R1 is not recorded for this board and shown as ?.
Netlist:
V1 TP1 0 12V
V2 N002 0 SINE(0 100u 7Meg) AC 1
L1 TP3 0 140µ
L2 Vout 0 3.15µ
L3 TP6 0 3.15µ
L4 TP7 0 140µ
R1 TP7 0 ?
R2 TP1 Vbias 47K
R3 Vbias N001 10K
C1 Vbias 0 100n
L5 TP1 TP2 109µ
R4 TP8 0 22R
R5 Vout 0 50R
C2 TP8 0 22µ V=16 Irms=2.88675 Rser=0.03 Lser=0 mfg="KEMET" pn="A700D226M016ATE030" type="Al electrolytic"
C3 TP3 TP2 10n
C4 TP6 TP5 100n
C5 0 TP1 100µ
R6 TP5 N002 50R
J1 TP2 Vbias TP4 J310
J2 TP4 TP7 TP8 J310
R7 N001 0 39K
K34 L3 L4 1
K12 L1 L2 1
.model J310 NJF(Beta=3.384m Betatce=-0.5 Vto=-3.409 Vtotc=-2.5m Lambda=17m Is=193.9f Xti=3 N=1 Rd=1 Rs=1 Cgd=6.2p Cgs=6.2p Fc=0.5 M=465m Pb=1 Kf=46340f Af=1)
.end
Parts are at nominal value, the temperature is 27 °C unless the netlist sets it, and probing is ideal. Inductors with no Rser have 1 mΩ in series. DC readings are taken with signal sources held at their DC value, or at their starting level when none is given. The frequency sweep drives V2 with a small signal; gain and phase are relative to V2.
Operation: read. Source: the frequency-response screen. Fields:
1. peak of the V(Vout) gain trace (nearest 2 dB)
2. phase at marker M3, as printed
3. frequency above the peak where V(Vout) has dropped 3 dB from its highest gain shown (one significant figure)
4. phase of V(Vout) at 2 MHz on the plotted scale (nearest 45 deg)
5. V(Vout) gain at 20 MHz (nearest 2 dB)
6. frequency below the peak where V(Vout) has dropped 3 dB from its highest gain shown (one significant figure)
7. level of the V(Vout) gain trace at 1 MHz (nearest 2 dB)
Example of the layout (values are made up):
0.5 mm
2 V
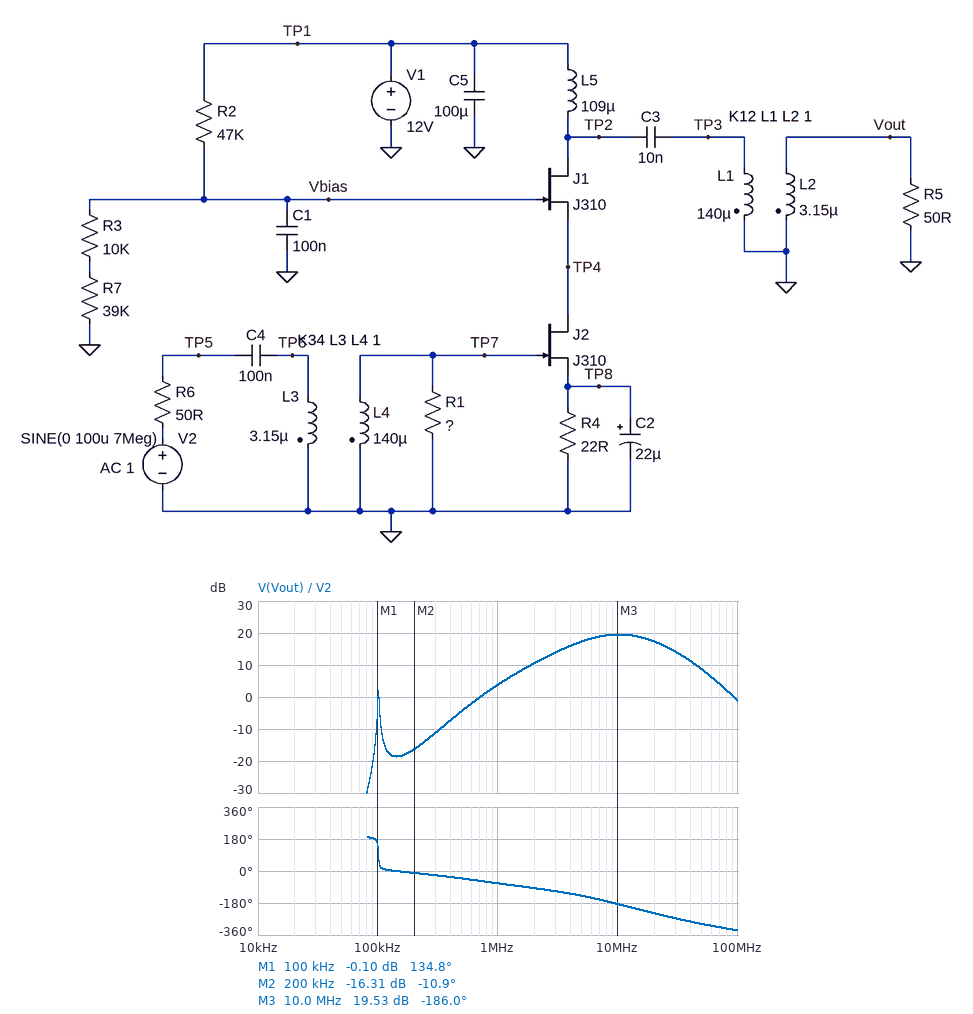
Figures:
20 dB
-186.0 deg
20 MHz
-90 deg
18 dB
4 MHz
4 dB
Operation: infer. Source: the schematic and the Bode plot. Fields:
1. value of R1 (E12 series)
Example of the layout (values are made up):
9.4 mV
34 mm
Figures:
680 Ω
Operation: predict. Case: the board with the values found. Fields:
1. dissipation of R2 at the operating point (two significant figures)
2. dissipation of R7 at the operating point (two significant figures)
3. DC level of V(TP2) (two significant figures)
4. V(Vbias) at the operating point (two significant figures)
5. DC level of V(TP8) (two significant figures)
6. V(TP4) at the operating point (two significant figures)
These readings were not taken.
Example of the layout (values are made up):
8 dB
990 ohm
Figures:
730 µW
610 µW
12 V
6.1 V
620 mV
6.7 V
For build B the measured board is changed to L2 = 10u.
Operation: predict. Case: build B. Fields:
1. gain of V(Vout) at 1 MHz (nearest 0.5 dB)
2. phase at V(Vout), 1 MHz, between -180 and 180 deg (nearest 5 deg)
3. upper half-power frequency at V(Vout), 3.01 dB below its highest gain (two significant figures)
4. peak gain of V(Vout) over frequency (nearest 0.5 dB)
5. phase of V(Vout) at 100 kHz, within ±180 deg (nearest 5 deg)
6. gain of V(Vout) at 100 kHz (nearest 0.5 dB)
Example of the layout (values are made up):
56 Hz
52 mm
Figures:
8.0 dB
-90 deg
30 MHz
15.0 dB
110 deg
-3.5 dB
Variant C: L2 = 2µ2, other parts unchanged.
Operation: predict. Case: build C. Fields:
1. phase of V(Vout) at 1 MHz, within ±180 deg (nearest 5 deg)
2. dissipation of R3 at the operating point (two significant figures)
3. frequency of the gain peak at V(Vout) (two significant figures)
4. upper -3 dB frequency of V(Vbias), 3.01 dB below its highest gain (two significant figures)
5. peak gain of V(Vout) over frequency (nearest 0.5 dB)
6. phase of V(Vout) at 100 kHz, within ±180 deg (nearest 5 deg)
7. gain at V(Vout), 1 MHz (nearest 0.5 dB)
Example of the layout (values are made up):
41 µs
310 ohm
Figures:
-65 deg
160 µW
11 MHz
20 MHz
21.0 dB
145 deg
2.5 dB
